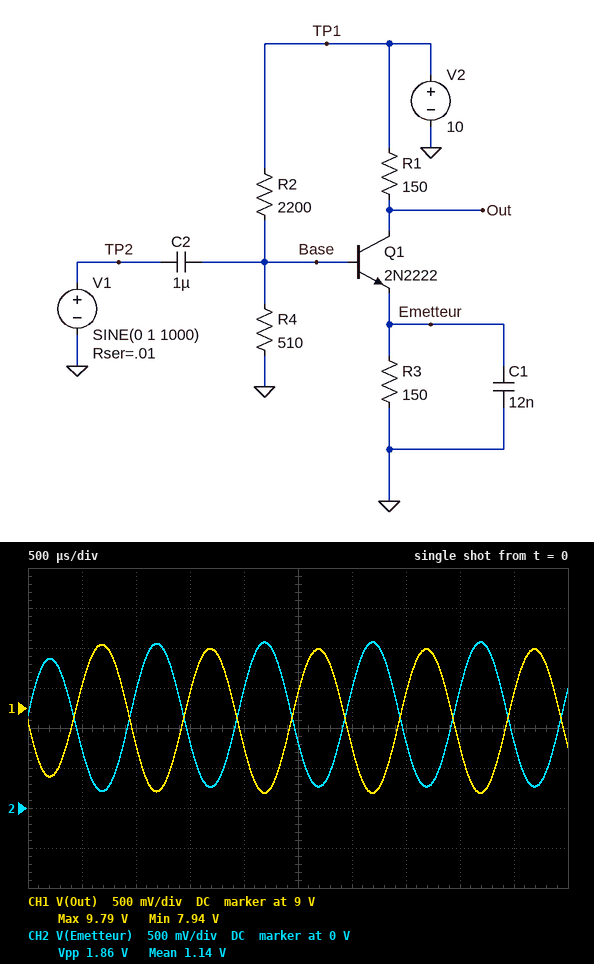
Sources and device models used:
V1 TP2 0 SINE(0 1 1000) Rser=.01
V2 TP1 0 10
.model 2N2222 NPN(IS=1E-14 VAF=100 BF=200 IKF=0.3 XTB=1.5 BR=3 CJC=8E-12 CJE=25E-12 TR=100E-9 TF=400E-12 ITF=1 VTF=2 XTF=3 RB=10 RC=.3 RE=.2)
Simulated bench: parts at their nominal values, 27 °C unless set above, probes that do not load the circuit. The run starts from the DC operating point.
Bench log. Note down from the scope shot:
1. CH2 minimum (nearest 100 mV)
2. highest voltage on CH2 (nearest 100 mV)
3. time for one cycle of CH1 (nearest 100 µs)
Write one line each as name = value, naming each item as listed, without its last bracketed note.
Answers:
CH2 minimum = 200 mV
highest voltage on CH2 = 2.1 V
time for one cycle of CH1 = 1.0 ms
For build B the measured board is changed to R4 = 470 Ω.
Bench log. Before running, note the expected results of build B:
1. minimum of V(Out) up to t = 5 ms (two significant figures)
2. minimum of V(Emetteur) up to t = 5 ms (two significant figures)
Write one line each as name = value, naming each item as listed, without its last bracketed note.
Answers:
minimum of V(Out) up to t = 5 ms = 8.1 V
minimum of V(Emetteur) up to t = 5 ms = 120 mV
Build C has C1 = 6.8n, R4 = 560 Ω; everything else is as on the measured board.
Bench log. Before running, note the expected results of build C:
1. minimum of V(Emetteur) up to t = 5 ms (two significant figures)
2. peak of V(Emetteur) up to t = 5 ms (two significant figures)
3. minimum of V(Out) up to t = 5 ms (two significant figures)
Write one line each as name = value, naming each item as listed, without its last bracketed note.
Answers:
minimum of V(Emetteur) up to t = 5 ms = 330 mV
peak of V(Emetteur) up to t = 5 ms = 2.2 V
minimum of V(Out) up to t = 5 ms = 7.8 V
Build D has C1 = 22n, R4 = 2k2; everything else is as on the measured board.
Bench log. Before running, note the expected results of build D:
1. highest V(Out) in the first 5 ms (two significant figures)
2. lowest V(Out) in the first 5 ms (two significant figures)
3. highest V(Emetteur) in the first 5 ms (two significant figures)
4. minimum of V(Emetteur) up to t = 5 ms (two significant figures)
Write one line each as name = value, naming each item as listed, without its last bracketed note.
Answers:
highest V(Out) in the first 5 ms = 7.0 V
lowest V(Out) in the first 5 ms = 5.1 V
highest V(Emetteur) in the first 5 ms = 5.0 V
minimum of V(Emetteur) up to t = 5 ms = 3.0 V
